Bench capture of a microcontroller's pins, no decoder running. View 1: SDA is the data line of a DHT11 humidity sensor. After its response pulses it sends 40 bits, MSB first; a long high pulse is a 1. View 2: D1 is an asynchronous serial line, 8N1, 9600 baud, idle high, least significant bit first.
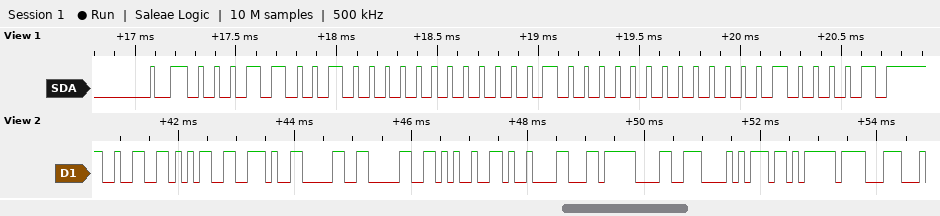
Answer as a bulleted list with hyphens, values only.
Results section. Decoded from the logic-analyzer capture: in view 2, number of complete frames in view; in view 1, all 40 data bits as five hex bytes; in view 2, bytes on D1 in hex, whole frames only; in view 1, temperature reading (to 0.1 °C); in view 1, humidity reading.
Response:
- 12
- 19 00 08 00 21
- 32 35 2E 30 30 25 09 EC 98 A8 EB 8F
- 8.0 °C
- 25 %
